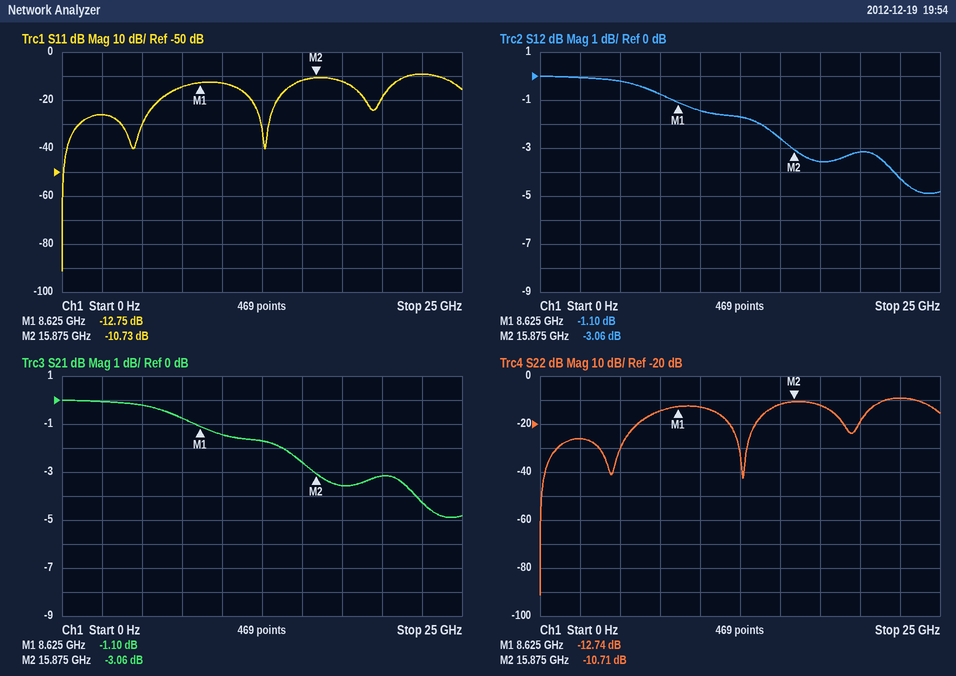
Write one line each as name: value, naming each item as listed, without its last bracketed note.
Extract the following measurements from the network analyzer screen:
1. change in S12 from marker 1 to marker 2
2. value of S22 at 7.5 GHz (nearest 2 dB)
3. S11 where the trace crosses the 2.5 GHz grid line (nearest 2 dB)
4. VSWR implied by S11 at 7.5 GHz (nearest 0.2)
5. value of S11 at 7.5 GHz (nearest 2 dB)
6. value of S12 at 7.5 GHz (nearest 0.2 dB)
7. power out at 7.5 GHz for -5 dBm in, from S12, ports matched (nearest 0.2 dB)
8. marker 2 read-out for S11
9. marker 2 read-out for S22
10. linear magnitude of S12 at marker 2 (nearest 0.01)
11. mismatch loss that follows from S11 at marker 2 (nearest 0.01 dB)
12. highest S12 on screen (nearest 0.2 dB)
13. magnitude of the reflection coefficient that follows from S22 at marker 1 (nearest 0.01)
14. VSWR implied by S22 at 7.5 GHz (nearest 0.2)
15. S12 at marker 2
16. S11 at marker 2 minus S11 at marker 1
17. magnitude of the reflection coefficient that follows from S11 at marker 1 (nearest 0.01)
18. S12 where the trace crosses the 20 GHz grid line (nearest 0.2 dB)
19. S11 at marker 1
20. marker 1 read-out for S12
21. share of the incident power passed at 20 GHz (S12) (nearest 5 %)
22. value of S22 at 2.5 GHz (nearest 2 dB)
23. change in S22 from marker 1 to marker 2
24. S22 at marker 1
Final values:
change in S12 from marker 1 to marker 2: -1.96 dB
value of S22 at 7.5 GHz: -14 dB
S11 where the trace crosses the 2.5 GHz grid line: -26 dB
VSWR implied by S11 at 7.5 GHz: 1.4
value of S11 at 7.5 GHz: -14 dB
value of S12 at 7.5 GHz: -0.8 dB
power out at 7.5 GHz for -5 dBm in, from S12, ports matched: -5.8 dBm
marker 2 read-out for S11: -10.73 dB
marker 2 read-out for S22: -10.71 dB
linear magnitude of S12 at marker 2: 0.70
mismatch loss that follows from S11 at marker 2: 0.38 dB
highest S12 on screen: 0.0 dB
magnitude of the reflection coefficient that follows from S22 at marker 1: 0.23
VSWR implied by S22 at 7.5 GHz: 1.4
S12 at marker 2: -3.06 dB
S11 at marker 2 minus S11 at marker 1: 2.02 dB
magnitude of the reflection coefficient that follows from S11 at marker 1: 0.23
S12 where the trace crosses the 20 GHz grid line: -3.2 dB
S11 at marker 1: -12.75 dB
marker 1 read-out for S12: -1.10 dB
share of the incident power passed at 20 GHz (S12): 50 %
value of S22 at 2.5 GHz: -26 dB
change in S22 from marker 1 to marker 2: 2.03 dB
S22 at marker 1: -12.74 dB
